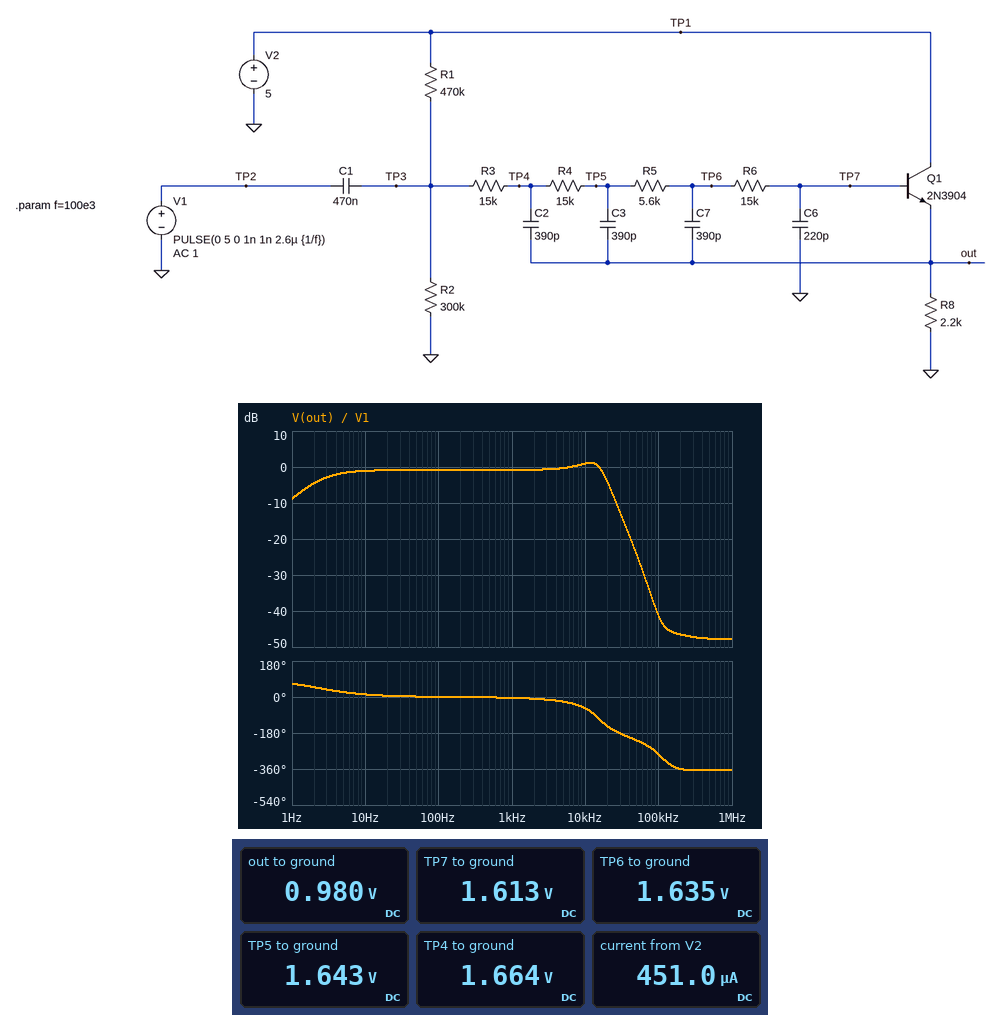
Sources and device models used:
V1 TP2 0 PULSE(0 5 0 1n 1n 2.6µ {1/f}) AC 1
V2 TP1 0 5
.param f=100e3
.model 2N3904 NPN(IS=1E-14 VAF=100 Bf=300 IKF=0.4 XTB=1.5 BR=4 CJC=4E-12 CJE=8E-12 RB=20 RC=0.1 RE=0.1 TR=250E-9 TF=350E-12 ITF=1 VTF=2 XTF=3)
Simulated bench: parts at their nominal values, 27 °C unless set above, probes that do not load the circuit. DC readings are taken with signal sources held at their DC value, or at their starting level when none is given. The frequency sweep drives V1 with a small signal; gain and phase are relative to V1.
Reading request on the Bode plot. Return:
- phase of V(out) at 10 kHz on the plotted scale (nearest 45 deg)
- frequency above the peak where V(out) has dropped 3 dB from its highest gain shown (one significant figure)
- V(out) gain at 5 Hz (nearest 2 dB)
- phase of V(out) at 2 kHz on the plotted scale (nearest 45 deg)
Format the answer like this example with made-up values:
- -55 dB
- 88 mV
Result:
- -45 deg
- 20 kHz
- -2 dB
- 0 deg
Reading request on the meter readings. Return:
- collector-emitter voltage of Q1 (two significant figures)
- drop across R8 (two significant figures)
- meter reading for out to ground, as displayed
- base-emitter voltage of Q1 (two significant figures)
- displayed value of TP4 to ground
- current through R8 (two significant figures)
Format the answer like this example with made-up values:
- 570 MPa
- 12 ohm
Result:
- 4.0 V
- 980 mV
- 0.980 V
- 630 mV
- 1.664 V
- 450 µA
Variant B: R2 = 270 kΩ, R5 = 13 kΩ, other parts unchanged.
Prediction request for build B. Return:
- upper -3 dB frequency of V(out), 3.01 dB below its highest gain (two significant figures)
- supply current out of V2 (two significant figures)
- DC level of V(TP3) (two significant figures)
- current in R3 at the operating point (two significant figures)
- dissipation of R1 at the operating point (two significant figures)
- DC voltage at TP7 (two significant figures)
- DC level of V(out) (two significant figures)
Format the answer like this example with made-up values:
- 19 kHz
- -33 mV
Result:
- 16 kHz
- 410 µA
- 1.6 V
- 1.3 µA
- 25 µW
- 1.5 V
- 890 mV
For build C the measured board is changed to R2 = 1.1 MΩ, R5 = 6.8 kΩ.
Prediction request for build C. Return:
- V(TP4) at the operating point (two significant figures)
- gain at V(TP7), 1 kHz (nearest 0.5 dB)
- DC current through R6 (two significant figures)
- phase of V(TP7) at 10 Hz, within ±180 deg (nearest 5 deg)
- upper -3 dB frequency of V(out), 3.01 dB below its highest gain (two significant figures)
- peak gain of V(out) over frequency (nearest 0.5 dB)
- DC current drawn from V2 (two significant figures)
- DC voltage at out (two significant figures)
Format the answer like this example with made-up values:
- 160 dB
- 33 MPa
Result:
- 2.6 V
- -0.5 dB
- 2.7 µA
- 10 deg
- 17 kHz
- 1.5 dB
- 830 µA
- 1.8 V
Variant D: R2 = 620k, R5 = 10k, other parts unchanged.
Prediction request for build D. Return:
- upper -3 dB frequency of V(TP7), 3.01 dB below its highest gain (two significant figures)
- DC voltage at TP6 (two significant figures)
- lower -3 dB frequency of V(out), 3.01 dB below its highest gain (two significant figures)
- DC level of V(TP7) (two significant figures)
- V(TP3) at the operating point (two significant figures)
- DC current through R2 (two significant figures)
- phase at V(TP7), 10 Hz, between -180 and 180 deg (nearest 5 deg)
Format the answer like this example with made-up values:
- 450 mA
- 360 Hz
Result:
- 17 kHz
- 2.2 V
- 3.9 Hz
- 2.1 V
- 2.3 V
- 3.6 µA
- 10 deg
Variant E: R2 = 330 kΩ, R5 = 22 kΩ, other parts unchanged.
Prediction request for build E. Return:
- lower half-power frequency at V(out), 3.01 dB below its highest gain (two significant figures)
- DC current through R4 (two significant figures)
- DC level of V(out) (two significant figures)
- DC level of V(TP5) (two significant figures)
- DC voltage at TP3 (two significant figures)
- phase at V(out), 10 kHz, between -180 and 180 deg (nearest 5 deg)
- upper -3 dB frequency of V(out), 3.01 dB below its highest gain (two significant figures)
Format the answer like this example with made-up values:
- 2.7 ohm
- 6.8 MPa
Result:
- 3.9 Hz
- 1.5 µA
- 1.0 V
- 1.7 V
- 1.8 V
- -80 deg
- 14 kHz
